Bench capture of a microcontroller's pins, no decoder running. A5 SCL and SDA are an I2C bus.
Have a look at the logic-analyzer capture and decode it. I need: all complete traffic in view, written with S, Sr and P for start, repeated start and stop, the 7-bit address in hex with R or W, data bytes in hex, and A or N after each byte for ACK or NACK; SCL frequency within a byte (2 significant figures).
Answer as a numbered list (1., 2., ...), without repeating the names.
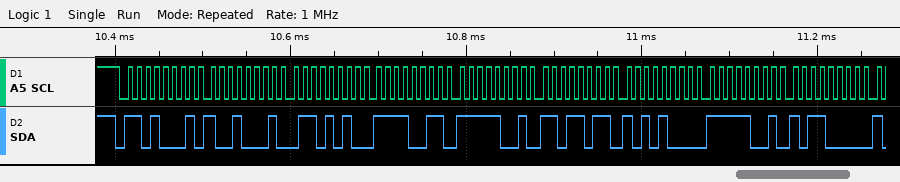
1. S 68R A 91 A 6A A F3 A F9 A DB A A8 A F9 A B0 A
2. 100 kHz
